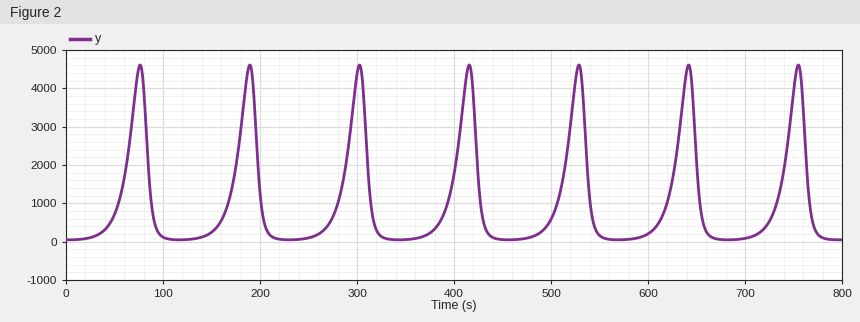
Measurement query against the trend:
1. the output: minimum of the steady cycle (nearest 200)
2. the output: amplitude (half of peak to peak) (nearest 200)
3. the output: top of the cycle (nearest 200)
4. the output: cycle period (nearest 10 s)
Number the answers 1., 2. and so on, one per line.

1. 0
2. 2200
3. 4600
4. 110 s
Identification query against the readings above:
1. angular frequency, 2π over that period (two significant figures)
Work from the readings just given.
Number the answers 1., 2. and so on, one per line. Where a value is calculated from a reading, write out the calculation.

1. 2π / 110 = 0.057 rad/s
